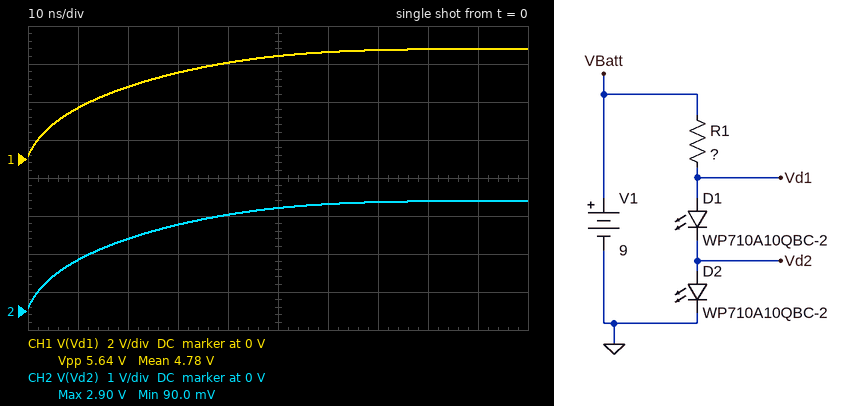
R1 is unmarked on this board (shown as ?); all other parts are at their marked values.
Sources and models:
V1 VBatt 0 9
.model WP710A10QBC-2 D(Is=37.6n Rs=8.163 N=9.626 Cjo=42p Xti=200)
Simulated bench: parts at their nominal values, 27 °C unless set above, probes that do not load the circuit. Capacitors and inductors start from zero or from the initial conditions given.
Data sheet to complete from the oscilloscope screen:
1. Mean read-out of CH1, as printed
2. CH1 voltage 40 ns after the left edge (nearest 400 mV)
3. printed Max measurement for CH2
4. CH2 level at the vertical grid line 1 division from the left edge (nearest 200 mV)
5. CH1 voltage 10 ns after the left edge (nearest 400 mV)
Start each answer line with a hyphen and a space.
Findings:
- 4.78 V
- 5.2 V
- 2.90 V
- 1.4 V
- 2.8 V
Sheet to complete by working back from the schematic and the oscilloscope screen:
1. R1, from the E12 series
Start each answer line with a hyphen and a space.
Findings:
- 820 Ω
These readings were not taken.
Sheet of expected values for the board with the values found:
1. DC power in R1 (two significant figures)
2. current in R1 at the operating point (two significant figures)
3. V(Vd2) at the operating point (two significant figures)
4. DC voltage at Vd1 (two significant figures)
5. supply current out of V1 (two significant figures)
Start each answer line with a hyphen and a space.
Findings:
- 12 mW
- 3.9 mA
- 2.9 V
- 5.8 V
- 3.9 mA
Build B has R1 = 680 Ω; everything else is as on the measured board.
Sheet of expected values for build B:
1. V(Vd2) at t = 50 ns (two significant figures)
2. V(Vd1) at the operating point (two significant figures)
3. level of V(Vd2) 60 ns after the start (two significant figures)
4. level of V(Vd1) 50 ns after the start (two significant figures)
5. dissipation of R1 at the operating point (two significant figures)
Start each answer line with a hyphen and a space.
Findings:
- 2.8 V
- 5.9 V
- 2.9 V
- 5.7 V
- 14 mW
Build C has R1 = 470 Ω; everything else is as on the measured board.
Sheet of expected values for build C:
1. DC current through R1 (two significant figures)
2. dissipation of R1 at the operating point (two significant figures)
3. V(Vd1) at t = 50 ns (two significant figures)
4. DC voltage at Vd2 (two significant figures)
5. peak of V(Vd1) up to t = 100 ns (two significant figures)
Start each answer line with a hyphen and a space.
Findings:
- 6.2 mA
- 18 mW
- 6.0 V
- 3.0 V
- 6.1 V
